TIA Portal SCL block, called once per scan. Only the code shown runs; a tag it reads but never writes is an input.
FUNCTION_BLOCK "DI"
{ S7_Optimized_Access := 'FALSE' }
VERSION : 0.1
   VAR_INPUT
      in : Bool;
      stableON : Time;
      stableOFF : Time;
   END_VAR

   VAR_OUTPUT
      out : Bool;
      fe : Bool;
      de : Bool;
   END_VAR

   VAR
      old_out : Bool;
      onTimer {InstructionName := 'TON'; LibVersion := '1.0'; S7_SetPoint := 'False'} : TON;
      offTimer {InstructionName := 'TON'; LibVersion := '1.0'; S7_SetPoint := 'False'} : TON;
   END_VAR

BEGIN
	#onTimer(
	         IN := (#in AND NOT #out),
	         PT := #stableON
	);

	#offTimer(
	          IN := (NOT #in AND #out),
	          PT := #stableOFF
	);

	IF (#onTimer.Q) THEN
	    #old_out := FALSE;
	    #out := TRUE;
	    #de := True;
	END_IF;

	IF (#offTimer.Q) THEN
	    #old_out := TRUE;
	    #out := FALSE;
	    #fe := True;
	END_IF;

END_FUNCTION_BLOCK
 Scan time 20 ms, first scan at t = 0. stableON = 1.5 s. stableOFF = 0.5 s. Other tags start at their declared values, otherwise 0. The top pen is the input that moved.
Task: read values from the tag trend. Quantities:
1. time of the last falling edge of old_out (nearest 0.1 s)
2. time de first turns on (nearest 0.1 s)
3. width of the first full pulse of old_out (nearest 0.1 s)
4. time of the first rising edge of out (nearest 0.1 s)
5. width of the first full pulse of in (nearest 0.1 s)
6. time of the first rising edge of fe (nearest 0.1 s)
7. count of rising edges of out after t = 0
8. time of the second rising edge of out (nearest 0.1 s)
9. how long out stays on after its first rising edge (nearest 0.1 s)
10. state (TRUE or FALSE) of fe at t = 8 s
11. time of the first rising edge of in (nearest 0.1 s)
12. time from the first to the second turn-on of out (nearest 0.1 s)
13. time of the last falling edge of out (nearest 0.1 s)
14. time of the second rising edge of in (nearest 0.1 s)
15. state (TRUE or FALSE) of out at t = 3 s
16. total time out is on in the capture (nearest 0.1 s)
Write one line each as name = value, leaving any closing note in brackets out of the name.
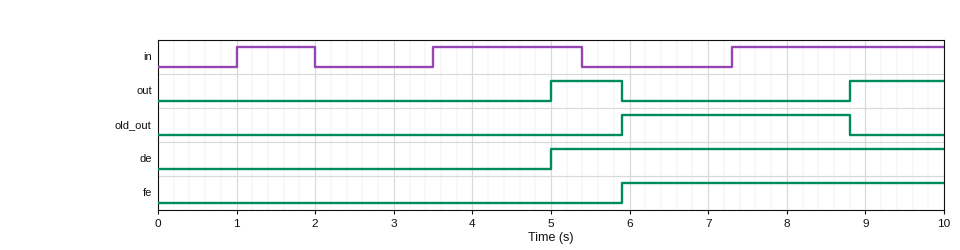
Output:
time of the last falling edge of old_out = 8.8 s
time de first turns on = 5.0 s
width of the first full pulse of old_out = 2.9 s
time of the first rising edge of out = 5.0 s
width of the first full pulse of in = 1.0 s
time of the first rising edge of fe = 5.9 s
count of rising edges of out after t = 0 = 2
time of the second rising edge of out = 8.8 s
how long out stays on after its first rising edge = 0.9 s
state (TRUE or FALSE) of fe at t = 8 s = TRUE
time of the first rising edge of in = 1.0 s
time from the first to the second turn-on of out = 3.8 s
time of the last falling edge of out = 5.9 s
time of the second rising edge of in = 3.5 s
state (TRUE or FALSE) of out at t = 3 s = FALSE
total time out is on in the capture = 2.1 s
